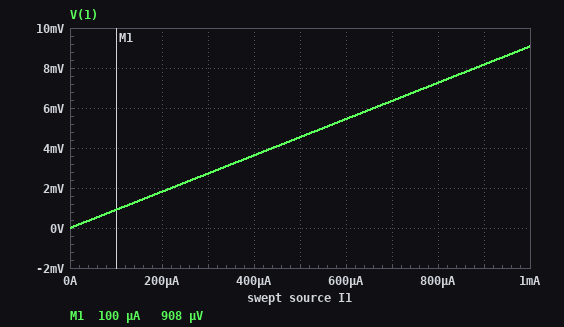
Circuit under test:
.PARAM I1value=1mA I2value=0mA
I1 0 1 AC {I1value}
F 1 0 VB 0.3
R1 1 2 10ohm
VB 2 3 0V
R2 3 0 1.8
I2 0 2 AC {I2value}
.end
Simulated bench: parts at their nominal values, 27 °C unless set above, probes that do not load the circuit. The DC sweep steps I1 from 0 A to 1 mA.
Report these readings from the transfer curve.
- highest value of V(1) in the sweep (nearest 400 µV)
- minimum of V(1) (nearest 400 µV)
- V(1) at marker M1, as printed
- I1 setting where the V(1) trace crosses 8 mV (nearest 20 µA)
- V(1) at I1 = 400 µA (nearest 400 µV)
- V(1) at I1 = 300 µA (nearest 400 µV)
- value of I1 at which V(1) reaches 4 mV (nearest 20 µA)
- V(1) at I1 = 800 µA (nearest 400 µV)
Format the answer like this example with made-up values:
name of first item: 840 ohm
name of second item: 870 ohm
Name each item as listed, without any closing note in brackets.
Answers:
highest value of V(1) in the sweep: 9.2 mV
minimum of V(1): 0 V
V(1) at marker M1, as printed: 908 µV
I1 setting where the V(1) trace crosses 8 mV: 880 µA
V(1) at I1 = 400 µA: 3.6 mV
V(1) at I1 = 300 µA: 2.8 mV
value of I1 at which V(1) reaches 4 mV: 440 µA
V(1) at I1 = 800 µA: 7.2 mV
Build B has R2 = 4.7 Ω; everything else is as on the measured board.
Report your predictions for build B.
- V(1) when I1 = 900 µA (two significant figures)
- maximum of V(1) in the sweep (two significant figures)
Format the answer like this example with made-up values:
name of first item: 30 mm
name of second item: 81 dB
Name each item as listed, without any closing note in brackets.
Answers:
V(1) when I1 = 900 µA: 10 mV
maximum of V(1) in the sweep: 11 mV
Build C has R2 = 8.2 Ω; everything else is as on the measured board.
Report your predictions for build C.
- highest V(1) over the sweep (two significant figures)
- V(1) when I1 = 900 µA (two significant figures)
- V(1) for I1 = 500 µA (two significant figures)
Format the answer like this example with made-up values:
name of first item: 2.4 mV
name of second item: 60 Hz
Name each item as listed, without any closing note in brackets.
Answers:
highest V(1) over the sweep: 14 mV
V(1) when I1 = 900 µA: 13 mV
V(1) for I1 = 500 µA: 7.0 mV
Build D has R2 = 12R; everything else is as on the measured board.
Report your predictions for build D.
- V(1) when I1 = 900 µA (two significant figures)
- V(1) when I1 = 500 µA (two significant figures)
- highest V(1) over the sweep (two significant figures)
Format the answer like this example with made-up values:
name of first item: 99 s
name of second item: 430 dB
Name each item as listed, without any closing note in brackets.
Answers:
V(1) when I1 = 900 µA: 15 mV
V(1) when I1 = 500 µA: 8.5 mV
highest V(1) over the sweep: 17 mV
